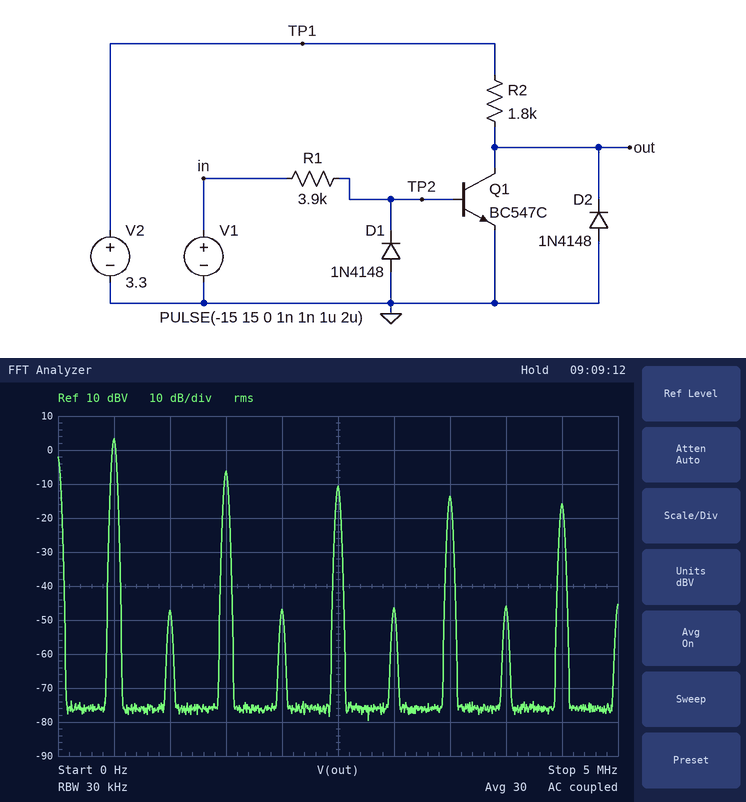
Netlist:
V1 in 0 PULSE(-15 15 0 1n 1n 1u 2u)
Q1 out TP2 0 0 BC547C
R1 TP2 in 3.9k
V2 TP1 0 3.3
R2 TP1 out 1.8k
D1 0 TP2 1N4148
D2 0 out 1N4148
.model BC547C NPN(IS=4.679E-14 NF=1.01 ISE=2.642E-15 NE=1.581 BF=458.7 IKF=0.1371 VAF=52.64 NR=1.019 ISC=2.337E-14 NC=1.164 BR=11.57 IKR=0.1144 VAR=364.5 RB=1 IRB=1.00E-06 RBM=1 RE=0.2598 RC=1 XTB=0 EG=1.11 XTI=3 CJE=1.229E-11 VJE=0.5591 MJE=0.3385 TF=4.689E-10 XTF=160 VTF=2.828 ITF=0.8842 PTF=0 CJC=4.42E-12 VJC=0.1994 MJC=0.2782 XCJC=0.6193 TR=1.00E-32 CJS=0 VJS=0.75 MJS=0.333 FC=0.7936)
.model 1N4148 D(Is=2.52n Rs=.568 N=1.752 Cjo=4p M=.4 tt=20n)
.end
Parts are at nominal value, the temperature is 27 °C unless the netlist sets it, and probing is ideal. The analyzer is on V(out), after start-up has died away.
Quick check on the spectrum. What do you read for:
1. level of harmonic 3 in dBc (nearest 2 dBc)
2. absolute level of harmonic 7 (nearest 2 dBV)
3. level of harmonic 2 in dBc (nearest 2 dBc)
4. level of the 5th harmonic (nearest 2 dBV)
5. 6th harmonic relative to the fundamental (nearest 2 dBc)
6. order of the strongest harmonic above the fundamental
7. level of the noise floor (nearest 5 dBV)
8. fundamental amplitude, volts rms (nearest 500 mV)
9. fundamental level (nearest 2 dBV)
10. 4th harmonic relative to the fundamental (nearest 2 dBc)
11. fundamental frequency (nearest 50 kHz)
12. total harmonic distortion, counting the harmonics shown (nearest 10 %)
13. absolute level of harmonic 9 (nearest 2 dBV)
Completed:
-10 dBc
-14 dBV
-50 dBc
-10 dBV
-50 dBc
3
-75 dBV
1.5 V
4 dBV
-50 dBc
500 kHz
40 %
-16 dBV
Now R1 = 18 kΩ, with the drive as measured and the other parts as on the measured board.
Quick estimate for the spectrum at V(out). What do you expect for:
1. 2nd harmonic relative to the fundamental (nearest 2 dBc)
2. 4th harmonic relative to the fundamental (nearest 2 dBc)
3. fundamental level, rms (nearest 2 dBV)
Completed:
-28 dBc
-28 dBc
4 dBV
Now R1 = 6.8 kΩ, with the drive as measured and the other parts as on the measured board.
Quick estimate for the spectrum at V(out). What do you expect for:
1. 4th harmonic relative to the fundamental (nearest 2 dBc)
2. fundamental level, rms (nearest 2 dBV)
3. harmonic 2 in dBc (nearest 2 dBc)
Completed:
-38 dBc
4 dBV
-38 dBc
